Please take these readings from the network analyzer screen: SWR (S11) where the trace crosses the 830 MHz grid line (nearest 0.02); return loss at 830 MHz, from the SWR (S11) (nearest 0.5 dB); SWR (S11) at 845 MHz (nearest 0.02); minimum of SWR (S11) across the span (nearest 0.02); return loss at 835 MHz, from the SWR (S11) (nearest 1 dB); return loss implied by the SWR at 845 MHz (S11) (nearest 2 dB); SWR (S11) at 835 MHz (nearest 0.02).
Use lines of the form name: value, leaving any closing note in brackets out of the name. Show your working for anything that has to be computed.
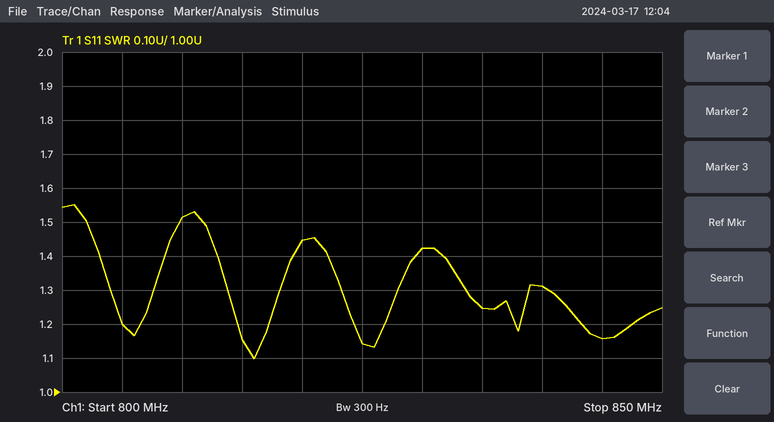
SWR (S11) where the trace crosses the 830 MHz grid line: 1.42
return loss at 830 MHz, from the SWR (S11): −20 log10((1.42 − 1)/(1.42 + 1)) ≈ 15.2 dB, so 15.0 dB to the nearest 0.5 dB
SWR (S11) at 845 MHz: 1.16
minimum of SWR (S11) across the span: 1.10
return loss at 835 MHz, from the SWR (S11): −20 log10((1.24 − 1)/(1.24 + 1)) ≈ 19 dB
return loss implied by the SWR at 845 MHz (S11): −20 log10((1.16 − 1)/(1.16 + 1)) ≈ 22.6 dB, so 22 dB to the nearest 2 dB
SWR (S11) at 835 MHz: 1.24
